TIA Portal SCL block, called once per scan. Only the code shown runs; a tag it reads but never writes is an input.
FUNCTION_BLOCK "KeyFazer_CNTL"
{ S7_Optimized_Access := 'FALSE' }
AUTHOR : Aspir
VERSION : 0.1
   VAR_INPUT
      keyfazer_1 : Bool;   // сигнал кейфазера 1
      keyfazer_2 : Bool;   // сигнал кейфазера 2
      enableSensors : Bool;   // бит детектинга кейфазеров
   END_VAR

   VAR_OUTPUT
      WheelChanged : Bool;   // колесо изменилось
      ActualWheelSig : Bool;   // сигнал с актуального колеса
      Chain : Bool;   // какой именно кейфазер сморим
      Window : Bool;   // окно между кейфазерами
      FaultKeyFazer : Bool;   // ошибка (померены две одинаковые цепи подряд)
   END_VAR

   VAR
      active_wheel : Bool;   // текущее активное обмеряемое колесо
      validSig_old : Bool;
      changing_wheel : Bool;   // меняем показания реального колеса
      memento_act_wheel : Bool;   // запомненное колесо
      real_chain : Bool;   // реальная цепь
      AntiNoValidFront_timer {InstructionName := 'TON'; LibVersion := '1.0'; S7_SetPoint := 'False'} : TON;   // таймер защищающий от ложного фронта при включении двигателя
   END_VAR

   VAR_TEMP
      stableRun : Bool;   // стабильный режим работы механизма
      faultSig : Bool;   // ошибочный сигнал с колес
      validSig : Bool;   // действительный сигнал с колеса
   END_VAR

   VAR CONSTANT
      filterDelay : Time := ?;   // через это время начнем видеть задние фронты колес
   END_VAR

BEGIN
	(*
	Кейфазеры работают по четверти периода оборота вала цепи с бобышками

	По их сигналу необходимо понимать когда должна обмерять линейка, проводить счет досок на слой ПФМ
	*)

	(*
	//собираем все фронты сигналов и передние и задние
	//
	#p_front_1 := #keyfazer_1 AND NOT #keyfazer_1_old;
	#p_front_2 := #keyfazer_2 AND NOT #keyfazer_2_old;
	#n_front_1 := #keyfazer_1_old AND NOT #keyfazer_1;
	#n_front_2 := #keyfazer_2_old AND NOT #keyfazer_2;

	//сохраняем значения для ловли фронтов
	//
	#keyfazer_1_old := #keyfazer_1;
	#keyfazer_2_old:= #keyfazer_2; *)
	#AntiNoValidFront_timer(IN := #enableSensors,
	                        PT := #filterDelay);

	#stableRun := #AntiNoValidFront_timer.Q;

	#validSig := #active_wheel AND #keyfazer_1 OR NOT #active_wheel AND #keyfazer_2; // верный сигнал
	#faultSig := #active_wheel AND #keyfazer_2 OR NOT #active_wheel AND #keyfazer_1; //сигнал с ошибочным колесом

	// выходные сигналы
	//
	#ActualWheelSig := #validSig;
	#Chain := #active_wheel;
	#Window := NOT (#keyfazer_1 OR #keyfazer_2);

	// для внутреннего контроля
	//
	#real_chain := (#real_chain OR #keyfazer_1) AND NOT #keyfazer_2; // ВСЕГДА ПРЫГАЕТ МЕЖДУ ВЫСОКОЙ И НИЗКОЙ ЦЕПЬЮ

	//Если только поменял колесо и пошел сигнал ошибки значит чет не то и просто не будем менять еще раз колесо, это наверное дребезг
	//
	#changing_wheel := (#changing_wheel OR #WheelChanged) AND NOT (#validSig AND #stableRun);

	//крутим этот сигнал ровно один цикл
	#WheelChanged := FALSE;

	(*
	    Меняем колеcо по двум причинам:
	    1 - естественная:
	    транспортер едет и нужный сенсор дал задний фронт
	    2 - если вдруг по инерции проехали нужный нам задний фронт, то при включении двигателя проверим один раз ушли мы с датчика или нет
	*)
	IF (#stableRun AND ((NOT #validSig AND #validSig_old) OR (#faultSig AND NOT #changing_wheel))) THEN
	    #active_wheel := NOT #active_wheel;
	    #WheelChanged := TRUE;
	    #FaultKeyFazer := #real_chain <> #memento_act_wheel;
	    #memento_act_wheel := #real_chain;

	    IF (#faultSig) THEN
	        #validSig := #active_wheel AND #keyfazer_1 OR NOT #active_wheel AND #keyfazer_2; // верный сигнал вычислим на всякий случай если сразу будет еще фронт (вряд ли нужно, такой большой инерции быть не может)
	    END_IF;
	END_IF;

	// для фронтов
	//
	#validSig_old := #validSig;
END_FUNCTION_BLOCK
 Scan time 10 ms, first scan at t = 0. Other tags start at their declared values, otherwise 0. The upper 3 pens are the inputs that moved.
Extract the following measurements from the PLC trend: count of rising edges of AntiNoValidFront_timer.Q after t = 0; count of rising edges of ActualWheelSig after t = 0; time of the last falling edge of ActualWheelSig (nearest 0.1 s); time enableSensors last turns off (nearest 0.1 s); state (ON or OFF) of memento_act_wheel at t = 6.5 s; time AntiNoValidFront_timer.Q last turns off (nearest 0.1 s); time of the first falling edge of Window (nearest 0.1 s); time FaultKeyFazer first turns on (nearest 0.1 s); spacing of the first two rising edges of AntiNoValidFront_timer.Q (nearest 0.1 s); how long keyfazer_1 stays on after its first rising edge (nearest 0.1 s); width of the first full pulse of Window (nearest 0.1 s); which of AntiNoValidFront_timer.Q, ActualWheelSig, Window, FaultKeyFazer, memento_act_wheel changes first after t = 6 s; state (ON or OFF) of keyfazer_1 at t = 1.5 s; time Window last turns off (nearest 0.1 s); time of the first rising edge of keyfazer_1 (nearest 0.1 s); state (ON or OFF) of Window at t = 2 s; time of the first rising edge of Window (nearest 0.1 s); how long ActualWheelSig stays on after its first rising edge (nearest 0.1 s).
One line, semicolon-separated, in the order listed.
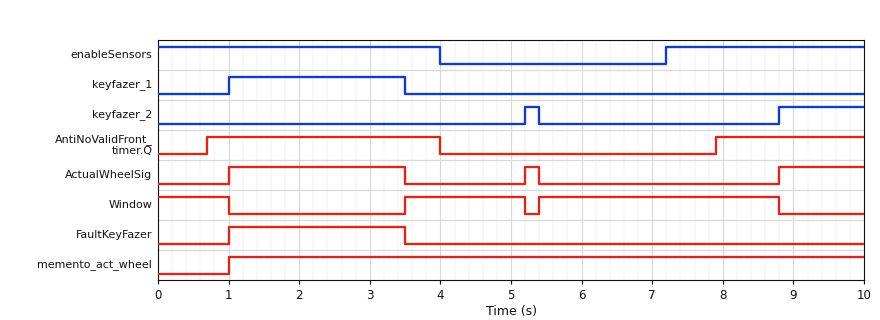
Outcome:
2; 3; 5.4 s; 4.0 s; ON; 4.0 s; 1.0 s; 1.0 s; 7.2 s; 2.5 s; 1.7 s; AntiNoValidFront_timer.Q; ON; 8.8 s; 1.0 s; OFF; 3.5 s; 2.5 s
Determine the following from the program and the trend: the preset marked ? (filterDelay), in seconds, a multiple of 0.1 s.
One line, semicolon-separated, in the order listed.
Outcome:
0.7 s
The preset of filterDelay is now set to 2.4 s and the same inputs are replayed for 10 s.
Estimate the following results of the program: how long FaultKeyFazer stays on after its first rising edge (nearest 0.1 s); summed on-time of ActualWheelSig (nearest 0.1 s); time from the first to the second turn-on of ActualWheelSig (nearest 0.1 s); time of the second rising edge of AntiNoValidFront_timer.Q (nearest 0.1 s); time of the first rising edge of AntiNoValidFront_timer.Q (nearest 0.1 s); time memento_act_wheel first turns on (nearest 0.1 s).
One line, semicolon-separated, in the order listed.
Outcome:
1.1 s; 2.5 s; 2.8 s; 9.6 s; 2.4 s; 2.4 s
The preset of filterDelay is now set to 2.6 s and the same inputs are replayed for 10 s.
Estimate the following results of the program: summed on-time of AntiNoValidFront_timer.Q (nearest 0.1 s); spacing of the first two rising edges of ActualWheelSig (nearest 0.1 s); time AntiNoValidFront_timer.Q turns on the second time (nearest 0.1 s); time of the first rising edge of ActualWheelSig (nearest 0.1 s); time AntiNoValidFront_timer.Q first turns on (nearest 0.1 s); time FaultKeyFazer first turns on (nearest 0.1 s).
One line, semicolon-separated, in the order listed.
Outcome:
1.6 s; 2.6 s; 9.8 s; 2.6 s; 2.6 s; 2.6 s
